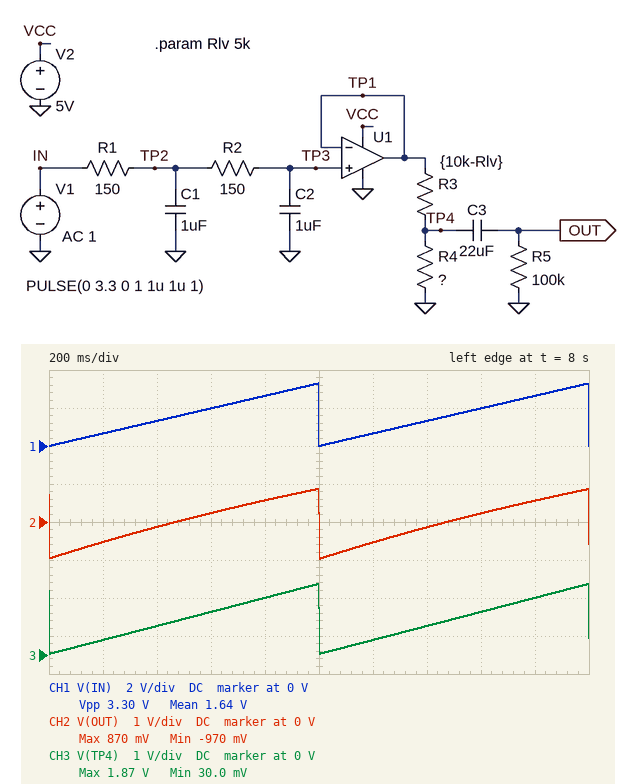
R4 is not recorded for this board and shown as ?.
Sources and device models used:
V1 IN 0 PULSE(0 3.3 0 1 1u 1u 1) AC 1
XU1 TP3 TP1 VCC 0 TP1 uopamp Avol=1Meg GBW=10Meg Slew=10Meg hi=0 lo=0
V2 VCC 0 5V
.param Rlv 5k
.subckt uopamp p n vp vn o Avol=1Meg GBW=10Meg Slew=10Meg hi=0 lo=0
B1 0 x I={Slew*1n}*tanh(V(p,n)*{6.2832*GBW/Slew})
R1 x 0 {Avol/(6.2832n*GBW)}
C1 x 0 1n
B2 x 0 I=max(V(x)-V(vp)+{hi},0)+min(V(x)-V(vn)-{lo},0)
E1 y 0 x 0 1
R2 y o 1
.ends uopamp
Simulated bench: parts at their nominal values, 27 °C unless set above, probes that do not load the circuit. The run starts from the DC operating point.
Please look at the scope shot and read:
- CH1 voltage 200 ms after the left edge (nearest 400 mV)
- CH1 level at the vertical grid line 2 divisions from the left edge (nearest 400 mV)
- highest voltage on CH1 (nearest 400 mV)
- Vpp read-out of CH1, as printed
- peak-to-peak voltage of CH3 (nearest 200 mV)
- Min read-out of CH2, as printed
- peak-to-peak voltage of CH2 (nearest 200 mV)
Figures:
800 mV
1.2 V
3.2 V
3.30 V
1.8 V
-970 mV
1.8 V
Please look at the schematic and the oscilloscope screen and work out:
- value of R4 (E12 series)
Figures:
6.8 kΩ
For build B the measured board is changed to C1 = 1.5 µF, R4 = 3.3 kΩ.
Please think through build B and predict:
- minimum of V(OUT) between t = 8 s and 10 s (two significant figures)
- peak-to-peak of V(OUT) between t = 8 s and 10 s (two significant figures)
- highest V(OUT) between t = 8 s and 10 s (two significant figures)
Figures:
-670 mV
1.3 V
610 mV
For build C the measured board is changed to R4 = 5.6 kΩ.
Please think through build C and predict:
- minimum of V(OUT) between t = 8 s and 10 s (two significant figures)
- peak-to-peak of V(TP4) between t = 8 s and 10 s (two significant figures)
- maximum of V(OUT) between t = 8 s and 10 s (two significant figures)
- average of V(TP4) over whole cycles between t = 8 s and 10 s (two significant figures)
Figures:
-890 mV
1.7 V
800 mV
870 mV
